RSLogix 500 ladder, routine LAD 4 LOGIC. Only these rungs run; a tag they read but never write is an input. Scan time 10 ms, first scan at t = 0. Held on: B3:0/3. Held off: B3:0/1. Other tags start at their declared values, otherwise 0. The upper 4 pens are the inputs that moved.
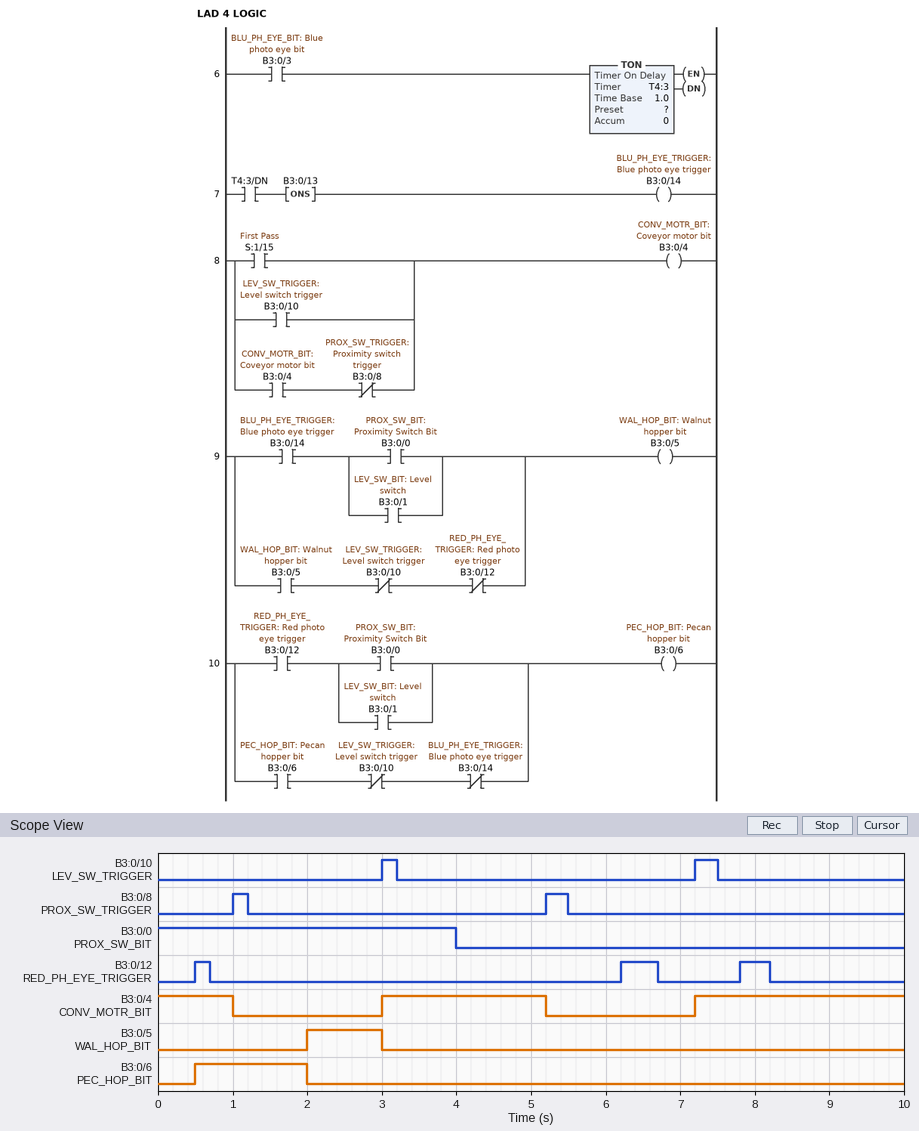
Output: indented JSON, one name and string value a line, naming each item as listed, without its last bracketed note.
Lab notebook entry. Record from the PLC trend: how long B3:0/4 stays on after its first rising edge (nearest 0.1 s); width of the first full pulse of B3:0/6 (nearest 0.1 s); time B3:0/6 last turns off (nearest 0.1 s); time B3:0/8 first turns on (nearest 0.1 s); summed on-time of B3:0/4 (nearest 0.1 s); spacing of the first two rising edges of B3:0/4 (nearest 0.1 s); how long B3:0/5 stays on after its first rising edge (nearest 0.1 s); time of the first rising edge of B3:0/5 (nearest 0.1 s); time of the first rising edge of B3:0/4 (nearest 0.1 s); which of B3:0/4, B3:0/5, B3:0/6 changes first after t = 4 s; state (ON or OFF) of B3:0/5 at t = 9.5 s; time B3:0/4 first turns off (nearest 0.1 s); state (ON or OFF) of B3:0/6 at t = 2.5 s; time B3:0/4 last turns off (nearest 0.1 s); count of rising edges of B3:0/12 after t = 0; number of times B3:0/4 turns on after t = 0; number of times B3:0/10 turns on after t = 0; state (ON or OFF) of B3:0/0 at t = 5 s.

{
  "how long B3:0/4 stays on after its first rising edge": "2.2 s",
  "width of the first full pulse of B3:0/6": "1.5 s",
  "time B3:0/6 last turns off": "2.0 s",
  "time B3:0/8 first turns on": "1.0 s",
  "summed on-time of B3:0/4": "6.0 s",
  "spacing of the first two rising edges of B3:0/4": "4.2 s",
  "how long B3:0/5 stays on after its first rising edge": "1.0 s",
  "time of the first rising edge of B3:0/5": "2.0 s",
  "time of the first rising edge of B3:0/4": "3.0 s",
  "which of B3:0/4, B3:0/5, B3:0/6 changes first after t = 4 s": "B3:0/4",
  "state (ON or OFF) of B3:0/5 at t = 9.5 s": "OFF",
  "time B3:0/4 first turns off": "1.0 s",
  "state (ON or OFF) of B3:0/6 at t = 2.5 s": "OFF",
  "time B3:0/4 last turns off": "5.2 s",
  "count of rising edges of B3:0/12 after t = 0": "3",
  "number of times B3:0/4 turns on after t = 0": "2",
  "number of times B3:0/10 turns on after t = 0": "2",
  "state (ON or OFF) of B3:0/0 at t = 5 s": "OFF"
}
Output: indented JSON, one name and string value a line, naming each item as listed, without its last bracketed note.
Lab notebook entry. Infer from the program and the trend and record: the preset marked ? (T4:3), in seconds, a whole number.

{
  "the preset marked ? (T4:3), in seconds, a whole number": "2 s"
}
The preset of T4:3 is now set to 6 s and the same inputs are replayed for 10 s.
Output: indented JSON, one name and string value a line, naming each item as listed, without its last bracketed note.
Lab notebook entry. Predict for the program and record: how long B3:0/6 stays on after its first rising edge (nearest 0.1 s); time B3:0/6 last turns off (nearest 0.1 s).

{
  "how long B3:0/6 stays on after its first rising edge": "2.5 s",
  "time B3:0/6 last turns off": "3.0 s"
}
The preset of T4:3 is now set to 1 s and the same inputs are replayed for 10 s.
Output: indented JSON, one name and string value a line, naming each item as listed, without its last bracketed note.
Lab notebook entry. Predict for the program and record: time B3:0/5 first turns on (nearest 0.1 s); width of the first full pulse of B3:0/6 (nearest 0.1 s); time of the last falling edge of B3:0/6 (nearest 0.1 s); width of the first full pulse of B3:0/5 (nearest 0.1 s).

{
  "time B3:0/5 first turns on": "1.0 s",
  "width of the first full pulse of B3:0/6": "0.5 s",
  "time of the last falling edge of B3:0/6": "1.0 s",
  "width of the first full pulse of B3:0/5": "2.0 s"
}
